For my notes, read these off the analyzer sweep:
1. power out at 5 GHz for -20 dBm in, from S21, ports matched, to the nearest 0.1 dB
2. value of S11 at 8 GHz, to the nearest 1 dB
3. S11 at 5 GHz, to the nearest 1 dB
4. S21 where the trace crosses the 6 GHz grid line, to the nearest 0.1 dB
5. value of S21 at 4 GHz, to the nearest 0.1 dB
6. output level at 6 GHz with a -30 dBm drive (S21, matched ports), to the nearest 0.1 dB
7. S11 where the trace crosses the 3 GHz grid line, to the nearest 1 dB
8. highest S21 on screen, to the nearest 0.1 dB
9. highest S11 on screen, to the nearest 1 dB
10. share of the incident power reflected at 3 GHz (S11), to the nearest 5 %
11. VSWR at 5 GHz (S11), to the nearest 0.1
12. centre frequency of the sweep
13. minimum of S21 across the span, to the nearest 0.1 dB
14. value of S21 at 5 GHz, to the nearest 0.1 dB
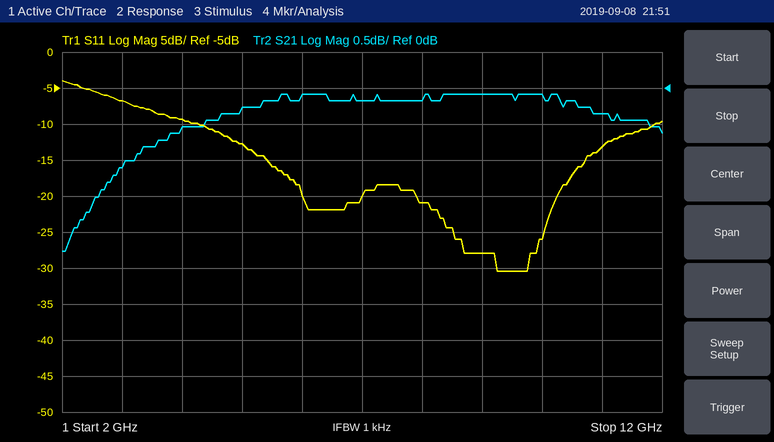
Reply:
-20.3 dBm
-21 dB
-13 dB
-0.1 dB
-0.5 dB
-30.1 dBm
-7 dB
-0.1 dB
-4 dB
20 %
1.6
7 GHz
-2.3 dB
-0.3 dB
